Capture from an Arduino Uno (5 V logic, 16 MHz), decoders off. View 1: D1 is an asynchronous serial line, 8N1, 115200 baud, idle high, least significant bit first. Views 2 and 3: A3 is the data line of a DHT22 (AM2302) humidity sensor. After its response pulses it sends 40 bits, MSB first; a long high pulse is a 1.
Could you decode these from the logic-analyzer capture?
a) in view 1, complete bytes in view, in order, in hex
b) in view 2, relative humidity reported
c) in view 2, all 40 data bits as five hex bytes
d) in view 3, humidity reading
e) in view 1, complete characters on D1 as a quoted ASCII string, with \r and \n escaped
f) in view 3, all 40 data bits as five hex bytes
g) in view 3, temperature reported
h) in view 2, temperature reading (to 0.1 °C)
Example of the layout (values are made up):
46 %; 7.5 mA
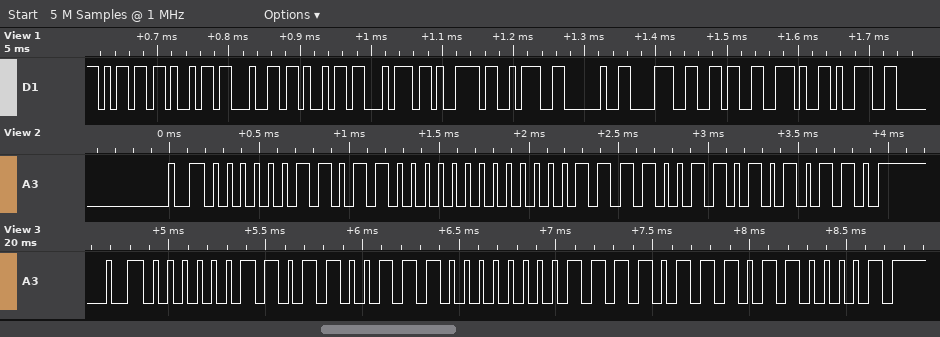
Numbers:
6D 69 64 69 74 79 3A 20 38 36 2E 39; 86.4 %; 03 60 00 F3 56; 87.1 %; "midity: 86.9"; 03 67 00 F7 61; 24.7 °C; 24.3 °C
